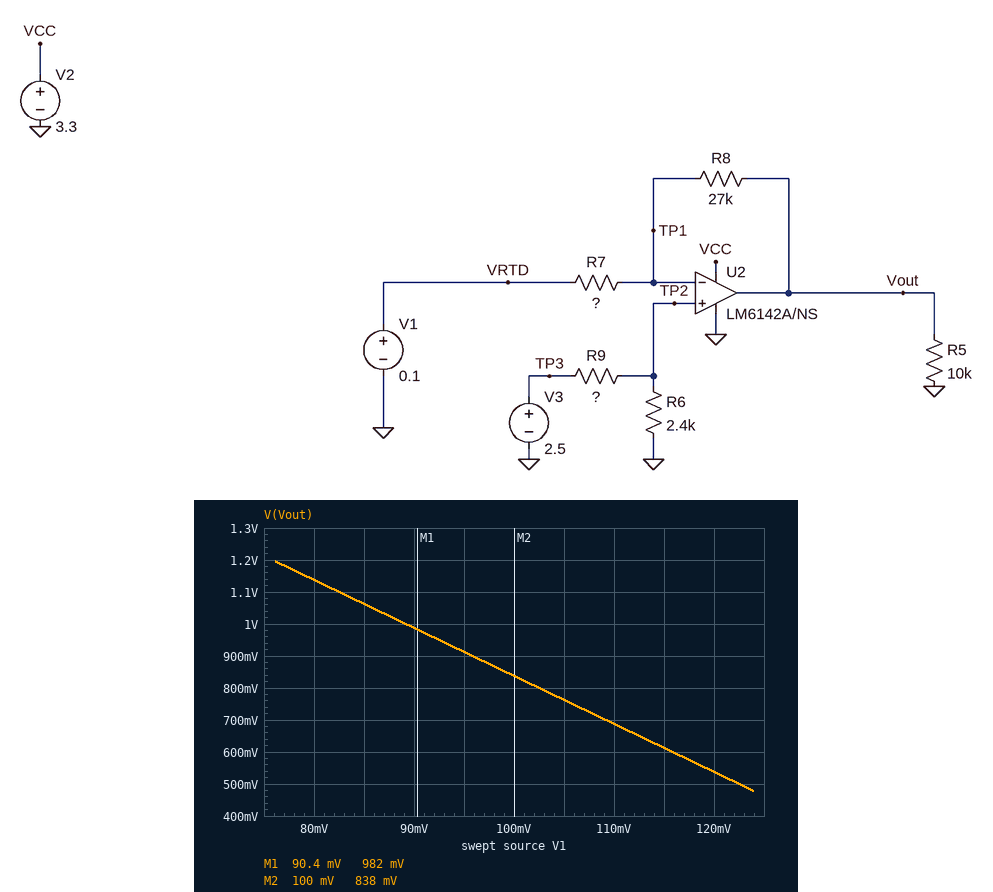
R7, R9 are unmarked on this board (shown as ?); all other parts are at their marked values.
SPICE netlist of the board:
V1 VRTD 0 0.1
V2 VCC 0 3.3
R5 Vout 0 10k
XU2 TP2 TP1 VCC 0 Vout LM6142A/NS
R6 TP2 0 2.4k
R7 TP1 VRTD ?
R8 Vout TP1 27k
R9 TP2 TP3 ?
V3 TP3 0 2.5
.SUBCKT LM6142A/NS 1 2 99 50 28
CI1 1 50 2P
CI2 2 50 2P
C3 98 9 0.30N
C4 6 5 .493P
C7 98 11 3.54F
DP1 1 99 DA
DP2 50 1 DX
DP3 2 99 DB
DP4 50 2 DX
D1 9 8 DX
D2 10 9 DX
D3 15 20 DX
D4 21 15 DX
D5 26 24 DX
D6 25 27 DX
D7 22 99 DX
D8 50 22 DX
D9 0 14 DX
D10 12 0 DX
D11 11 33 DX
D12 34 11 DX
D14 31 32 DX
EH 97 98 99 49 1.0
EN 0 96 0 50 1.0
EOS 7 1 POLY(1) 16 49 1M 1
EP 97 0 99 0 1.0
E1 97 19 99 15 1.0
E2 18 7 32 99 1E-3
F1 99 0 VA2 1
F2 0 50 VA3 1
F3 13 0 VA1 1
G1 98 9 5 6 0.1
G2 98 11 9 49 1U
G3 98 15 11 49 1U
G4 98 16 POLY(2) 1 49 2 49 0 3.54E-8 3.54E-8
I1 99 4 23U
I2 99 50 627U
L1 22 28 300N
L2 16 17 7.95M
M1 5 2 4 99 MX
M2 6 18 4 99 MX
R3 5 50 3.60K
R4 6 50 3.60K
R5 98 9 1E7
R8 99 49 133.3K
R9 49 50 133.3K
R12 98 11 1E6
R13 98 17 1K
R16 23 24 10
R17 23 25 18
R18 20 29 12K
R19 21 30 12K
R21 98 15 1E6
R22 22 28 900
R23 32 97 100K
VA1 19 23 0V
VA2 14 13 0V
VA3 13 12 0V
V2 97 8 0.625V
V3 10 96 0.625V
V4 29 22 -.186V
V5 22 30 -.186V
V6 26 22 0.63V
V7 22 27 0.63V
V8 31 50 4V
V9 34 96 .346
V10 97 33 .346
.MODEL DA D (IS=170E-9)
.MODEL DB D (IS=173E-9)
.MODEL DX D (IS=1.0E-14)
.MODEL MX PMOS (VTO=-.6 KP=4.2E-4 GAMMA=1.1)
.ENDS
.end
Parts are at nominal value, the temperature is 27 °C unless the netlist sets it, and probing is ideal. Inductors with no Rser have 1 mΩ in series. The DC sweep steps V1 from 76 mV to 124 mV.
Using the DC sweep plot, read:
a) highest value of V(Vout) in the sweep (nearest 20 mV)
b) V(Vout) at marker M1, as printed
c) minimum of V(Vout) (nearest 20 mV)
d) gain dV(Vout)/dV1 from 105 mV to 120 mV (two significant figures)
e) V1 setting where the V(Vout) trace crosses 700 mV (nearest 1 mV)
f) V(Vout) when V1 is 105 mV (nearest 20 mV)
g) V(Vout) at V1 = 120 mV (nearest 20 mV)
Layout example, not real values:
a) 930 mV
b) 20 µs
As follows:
a) 1.20 V
b) 982 mV
c) 480 mV
d) -15 V/V
e) 109 mV
f) 760 mV
g) 540 mV
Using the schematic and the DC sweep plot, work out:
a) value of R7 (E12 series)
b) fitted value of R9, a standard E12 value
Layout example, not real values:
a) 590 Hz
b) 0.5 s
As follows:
a) 1.8 kΩ
b) 39 kΩ
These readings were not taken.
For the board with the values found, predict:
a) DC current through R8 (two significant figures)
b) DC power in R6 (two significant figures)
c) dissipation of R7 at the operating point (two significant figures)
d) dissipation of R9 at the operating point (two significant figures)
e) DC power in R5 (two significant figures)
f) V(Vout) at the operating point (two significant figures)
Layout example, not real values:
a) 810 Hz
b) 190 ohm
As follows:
a) 26 µA
b) 8.8 µW
c) 1.2 µW
d) 140 µW
e) 70 µW
f) 840 mV
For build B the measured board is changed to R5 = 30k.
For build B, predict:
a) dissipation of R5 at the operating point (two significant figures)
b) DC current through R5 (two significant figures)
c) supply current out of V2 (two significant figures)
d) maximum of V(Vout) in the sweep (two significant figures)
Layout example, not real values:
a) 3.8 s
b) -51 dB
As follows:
a) 23 µW
b) 28 µA
c) 720 µA
d) 1.2 V
